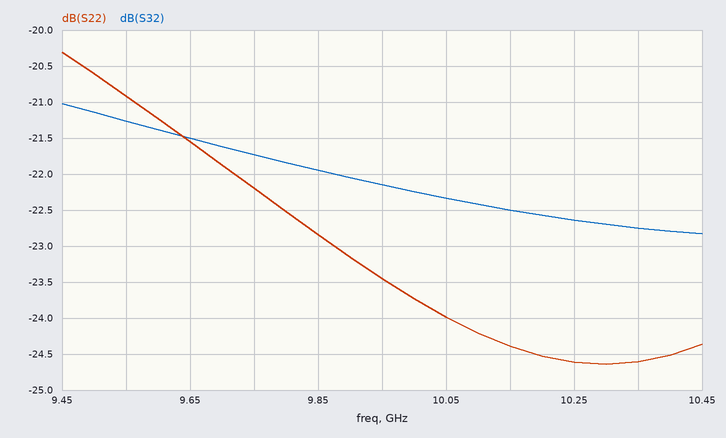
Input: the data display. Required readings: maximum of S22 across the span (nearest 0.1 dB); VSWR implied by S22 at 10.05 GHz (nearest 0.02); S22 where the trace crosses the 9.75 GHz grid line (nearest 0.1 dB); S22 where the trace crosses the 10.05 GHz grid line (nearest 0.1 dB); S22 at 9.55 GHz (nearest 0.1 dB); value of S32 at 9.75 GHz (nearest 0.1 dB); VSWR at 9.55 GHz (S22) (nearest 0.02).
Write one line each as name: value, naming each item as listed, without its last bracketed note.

maximum of S22 across the span: -20.3 dB
VSWR implied by S22 at 10.05 GHz: 1.14
S22 where the trace crosses the 9.75 GHz grid line: -22.2 dB
S22 where the trace crosses the 10.05 GHz grid line: -24.0 dB
S22 at 9.55 GHz: -20.9 dB
value of S32 at 9.75 GHz: -21.7 dB
VSWR at 9.55 GHz (S22): 1.20
